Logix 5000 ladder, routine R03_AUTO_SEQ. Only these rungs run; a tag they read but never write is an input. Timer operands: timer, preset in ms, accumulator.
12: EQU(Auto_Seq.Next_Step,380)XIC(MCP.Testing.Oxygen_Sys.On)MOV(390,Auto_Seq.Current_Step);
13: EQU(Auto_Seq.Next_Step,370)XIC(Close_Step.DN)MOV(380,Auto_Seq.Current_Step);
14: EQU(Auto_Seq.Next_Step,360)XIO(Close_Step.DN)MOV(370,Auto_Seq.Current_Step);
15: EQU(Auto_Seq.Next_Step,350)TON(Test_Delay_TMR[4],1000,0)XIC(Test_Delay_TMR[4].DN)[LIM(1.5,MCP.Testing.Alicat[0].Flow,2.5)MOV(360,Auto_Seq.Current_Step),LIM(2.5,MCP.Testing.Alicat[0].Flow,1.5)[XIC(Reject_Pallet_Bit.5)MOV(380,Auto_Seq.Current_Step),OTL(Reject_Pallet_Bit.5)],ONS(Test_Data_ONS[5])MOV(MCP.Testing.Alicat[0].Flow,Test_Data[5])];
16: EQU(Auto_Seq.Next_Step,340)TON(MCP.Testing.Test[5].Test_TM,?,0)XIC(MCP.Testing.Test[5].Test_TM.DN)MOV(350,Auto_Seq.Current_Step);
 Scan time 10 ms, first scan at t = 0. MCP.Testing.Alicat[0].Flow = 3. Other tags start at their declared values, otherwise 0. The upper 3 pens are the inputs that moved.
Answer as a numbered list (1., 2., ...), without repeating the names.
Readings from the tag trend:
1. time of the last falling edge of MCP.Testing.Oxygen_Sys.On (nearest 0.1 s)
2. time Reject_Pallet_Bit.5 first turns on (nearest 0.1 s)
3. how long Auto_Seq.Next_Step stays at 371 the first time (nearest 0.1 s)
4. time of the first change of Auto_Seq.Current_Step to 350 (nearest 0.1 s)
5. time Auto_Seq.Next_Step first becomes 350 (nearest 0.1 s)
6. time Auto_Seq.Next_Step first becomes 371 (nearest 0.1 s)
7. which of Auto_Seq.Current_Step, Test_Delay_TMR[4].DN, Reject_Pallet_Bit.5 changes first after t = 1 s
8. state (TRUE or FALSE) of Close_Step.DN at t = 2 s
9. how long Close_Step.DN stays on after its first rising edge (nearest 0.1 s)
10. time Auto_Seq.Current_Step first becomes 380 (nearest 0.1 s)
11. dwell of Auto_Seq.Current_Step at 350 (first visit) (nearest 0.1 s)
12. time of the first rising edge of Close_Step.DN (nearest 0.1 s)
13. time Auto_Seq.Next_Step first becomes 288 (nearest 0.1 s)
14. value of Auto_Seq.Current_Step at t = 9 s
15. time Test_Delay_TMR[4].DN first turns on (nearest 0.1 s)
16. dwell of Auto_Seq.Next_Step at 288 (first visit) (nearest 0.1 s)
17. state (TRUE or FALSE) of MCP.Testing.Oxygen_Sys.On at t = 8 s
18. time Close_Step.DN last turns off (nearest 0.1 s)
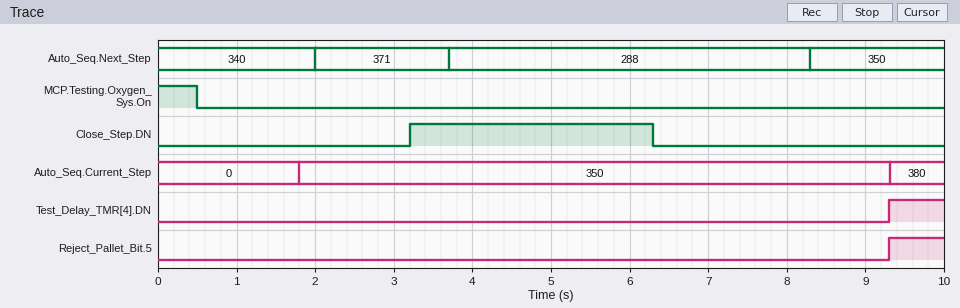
1. 0.5 s
2. 9.3 s
3. 1.7 s
4. 1.8 s
5. 8.3 s
6. 2.0 s
7. Auto_Seq.Current_Step
8. FALSE
9. 3.1 s
10. 9.3 s
11. 7.5 s
12. 3.2 s
13. 3.7 s
14. 350
15. 9.3 s
16. 4.6 s
17. FALSE
18. 6.3 s
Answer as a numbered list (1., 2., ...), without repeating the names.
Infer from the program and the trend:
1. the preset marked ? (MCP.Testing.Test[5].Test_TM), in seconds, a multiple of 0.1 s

1. 1.8 s
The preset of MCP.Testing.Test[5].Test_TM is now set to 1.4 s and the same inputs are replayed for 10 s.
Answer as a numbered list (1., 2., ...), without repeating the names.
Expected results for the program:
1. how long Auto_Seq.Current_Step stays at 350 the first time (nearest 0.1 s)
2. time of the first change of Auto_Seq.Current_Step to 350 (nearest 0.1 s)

1. 7.9 s
2. 1.4 s
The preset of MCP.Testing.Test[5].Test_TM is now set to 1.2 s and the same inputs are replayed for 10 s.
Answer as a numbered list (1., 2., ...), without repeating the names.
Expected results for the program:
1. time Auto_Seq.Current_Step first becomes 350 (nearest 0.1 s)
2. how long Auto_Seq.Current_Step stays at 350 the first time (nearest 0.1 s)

1. 1.2 s
2. 8.1 s
